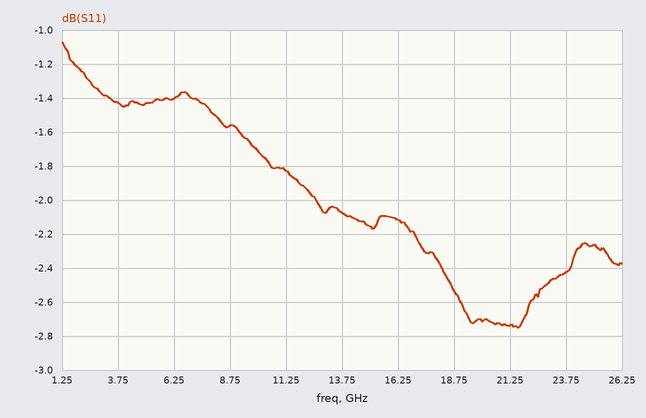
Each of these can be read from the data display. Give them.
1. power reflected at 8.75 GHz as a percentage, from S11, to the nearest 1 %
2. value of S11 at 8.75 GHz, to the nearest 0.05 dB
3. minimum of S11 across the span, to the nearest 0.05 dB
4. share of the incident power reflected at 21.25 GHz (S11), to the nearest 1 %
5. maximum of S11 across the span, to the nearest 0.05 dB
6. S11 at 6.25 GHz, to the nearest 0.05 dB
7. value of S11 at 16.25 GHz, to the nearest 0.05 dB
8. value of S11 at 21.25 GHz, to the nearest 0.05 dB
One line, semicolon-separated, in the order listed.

70 %; -1.55 dB; -2.75 dB; 53 %; -1.05 dB; -1.40 dB; -2.10 dB; -2.75 dB
